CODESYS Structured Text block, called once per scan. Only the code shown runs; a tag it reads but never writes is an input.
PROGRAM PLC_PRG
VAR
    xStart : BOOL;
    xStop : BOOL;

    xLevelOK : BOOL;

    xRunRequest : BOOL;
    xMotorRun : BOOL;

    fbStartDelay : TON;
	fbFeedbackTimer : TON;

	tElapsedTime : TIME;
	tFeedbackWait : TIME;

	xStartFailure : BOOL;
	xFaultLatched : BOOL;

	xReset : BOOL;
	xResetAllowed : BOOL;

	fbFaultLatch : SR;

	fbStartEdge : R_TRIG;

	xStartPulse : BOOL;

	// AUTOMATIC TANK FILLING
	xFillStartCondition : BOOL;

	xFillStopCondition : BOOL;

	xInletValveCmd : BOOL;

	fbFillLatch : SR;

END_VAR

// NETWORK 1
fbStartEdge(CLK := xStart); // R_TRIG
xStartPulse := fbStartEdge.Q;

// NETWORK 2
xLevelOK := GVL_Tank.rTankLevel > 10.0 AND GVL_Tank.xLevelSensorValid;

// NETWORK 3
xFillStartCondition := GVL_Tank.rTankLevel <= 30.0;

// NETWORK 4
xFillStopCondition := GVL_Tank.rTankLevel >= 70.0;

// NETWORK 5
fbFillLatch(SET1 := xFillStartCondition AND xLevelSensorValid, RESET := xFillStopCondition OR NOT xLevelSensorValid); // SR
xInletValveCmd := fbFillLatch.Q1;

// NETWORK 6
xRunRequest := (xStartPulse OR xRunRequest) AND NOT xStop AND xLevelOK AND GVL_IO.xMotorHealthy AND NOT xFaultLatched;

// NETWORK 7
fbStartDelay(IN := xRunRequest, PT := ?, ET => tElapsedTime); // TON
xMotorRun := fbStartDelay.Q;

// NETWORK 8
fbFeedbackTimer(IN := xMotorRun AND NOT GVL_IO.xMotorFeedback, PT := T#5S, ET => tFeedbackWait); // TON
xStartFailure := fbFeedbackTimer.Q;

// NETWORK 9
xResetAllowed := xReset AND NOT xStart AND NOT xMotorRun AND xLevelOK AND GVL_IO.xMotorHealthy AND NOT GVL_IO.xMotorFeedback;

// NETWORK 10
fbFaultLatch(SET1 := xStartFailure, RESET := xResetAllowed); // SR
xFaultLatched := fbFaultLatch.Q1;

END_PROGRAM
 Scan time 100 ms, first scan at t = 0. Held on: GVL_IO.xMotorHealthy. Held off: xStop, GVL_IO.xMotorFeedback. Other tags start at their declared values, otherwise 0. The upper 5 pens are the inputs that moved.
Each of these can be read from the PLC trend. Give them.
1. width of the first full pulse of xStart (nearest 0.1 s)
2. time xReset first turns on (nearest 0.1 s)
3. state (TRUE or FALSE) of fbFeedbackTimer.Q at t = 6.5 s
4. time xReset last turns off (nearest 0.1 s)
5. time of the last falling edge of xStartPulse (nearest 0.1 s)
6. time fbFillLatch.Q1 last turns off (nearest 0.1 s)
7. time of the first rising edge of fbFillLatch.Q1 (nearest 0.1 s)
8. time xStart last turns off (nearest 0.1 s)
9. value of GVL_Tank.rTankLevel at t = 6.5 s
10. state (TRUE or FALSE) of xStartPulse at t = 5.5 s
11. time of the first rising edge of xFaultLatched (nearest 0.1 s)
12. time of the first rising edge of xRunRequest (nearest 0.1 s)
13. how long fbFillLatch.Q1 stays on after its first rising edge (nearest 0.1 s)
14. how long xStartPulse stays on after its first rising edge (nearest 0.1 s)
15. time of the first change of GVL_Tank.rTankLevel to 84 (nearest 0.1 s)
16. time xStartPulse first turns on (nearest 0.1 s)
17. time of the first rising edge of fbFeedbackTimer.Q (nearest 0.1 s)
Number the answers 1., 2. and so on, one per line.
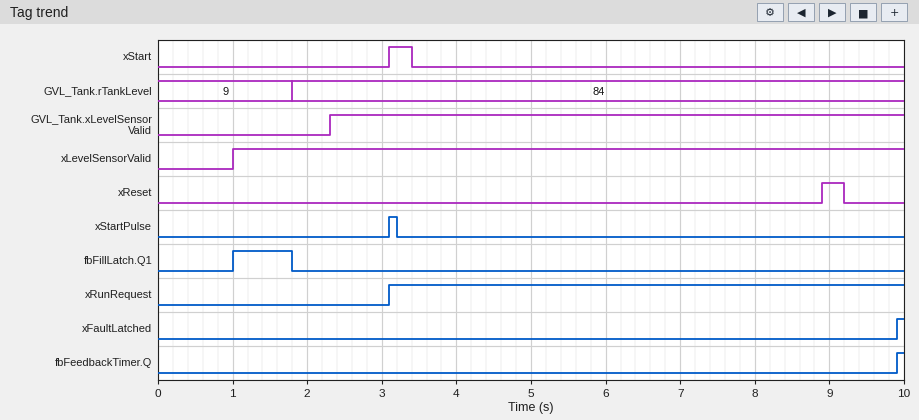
1. 0.3 s
2. 8.9 s
3. FALSE
4. 9.2 s
5. 3.2 s
6. 1.8 s
7. 1.0 s
8. 3.4 s
9. 84
10. FALSE
11. 9.9 s
12. 3.1 s
13. 0.8 s
14. 0.1 s
15. 1.8 s
16. 3.1 s
17. 9.9 s
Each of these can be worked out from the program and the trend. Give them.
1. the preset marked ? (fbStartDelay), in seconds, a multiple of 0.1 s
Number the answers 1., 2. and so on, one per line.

1. 1.8 s
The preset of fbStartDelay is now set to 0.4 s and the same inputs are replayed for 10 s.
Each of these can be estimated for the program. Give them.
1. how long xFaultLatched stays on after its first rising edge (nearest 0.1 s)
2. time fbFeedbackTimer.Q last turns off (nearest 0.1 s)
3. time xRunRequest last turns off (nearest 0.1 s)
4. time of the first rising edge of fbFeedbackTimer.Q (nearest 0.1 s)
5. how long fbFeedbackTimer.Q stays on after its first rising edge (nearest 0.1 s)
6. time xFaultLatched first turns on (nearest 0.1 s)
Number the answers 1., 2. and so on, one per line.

1. 0.4 s
2. 8.6 s
3. 8.6 s
4. 8.5 s
5. 0.1 s
6. 8.5 s
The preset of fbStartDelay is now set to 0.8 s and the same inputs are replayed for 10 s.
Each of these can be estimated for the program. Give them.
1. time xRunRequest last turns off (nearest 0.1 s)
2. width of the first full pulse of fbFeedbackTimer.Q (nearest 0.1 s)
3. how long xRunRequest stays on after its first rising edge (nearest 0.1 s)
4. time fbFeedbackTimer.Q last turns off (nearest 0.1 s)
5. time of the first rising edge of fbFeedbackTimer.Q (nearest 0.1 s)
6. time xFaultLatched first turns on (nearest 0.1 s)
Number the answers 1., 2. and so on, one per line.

1. 9.0 s
2. 0.1 s
3. 5.9 s
4. 9.0 s
5. 8.9 s
6. 8.9 s
